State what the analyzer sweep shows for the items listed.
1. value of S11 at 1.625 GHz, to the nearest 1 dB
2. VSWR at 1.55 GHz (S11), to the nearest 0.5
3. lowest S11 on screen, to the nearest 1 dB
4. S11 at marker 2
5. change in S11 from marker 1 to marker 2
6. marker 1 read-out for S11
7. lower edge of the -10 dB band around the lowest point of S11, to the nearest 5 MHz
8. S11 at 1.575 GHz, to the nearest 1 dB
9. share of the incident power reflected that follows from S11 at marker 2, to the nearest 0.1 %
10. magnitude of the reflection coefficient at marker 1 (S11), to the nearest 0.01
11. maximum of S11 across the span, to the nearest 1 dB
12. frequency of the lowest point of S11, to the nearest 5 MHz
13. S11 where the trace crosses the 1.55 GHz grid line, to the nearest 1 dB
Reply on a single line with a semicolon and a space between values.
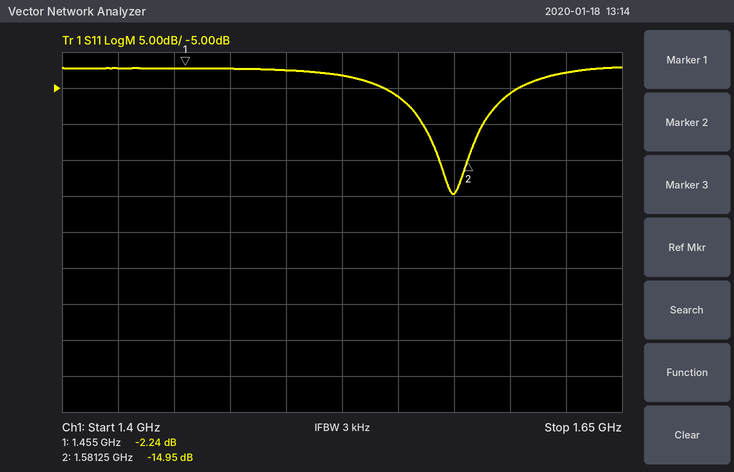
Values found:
-3 dB; 3.0; -20 dB; -14.95 dB; -12.71 dB; -2.24 dB; 1.560 GHz; -20 dB; 3.2 %; 0.77; -2 dB; 1.575 GHz; -6 dB
